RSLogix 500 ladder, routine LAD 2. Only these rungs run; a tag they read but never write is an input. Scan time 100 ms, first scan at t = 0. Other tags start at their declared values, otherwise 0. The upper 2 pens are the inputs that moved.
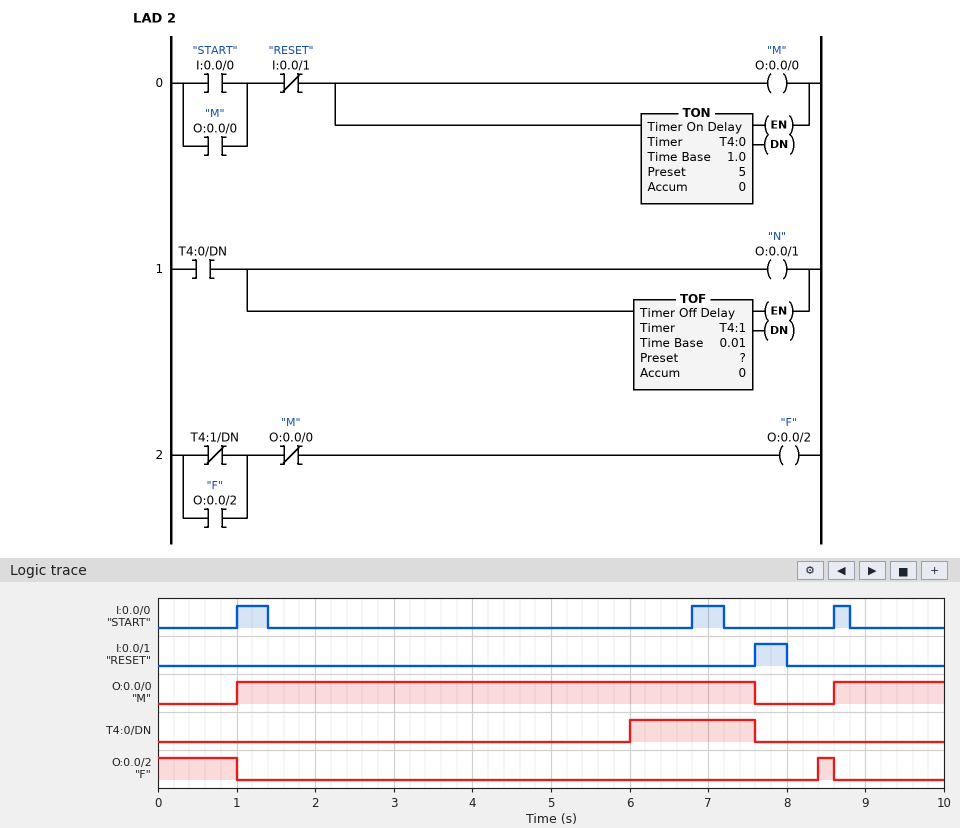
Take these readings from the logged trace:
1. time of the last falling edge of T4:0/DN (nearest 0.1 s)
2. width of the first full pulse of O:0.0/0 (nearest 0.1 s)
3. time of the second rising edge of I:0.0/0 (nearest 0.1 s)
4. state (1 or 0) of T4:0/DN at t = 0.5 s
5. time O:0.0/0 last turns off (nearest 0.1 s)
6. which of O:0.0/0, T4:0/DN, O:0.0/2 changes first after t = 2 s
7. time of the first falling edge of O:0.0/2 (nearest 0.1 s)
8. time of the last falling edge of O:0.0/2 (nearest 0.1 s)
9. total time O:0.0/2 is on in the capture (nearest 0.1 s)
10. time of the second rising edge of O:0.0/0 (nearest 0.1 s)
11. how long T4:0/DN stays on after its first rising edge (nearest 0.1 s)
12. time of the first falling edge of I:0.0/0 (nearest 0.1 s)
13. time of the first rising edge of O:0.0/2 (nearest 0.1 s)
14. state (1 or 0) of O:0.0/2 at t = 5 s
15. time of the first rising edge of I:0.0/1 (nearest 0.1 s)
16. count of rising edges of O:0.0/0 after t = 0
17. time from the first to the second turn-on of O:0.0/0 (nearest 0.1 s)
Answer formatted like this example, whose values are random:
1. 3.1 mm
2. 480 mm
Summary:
1. 7.6 s
2. 6.6 s
3. 6.8 s
4. 0
5. 7.6 s
6. T4:0/DN
7. 1.0 s
8. 8.6 s
9. 1.2 s
10. 8.6 s
11. 1.6 s
12. 1.4 s
13. 8.4 s
14. 0
15. 7.6 s
16. 2
17. 7.6 s
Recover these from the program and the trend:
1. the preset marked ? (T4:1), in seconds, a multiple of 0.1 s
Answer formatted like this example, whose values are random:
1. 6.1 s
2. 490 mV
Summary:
1. 0.8 s
